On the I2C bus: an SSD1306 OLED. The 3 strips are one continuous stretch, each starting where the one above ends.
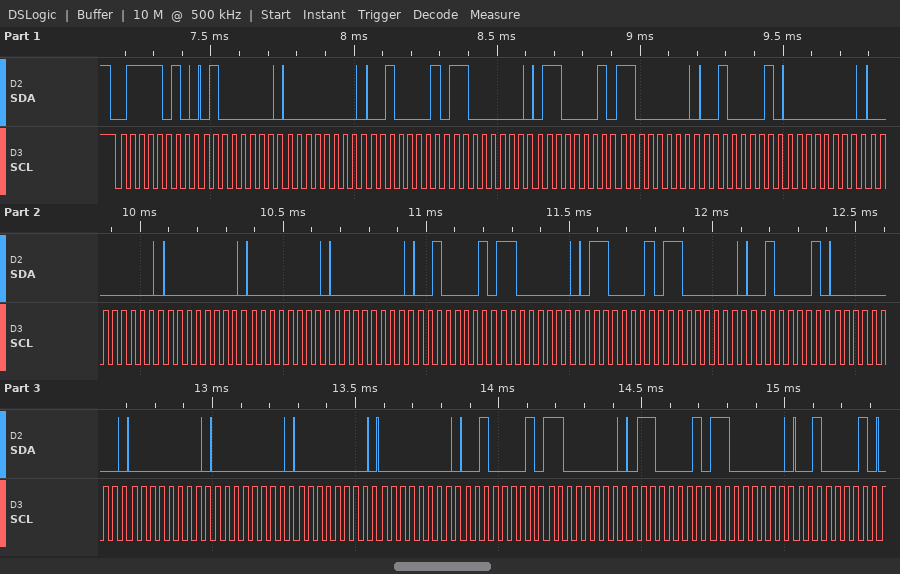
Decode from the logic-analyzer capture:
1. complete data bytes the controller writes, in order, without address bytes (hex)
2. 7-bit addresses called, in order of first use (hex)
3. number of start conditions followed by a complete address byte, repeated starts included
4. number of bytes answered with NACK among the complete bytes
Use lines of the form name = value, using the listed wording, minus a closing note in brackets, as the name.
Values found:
complete data bytes the controller writes, in order, without address bytes = 40 00 21 C0 61 C0 21 00 00 00 00 00 21 C0 61 C0 21 00 00 00 00 00 21 C0 61 C0 21
7-bit addresses called, in order of first use = 0x3D
number of start conditions followed by a complete address byte, repeated starts included = 1
number of bytes answered with NACK among the complete bytes = 0
